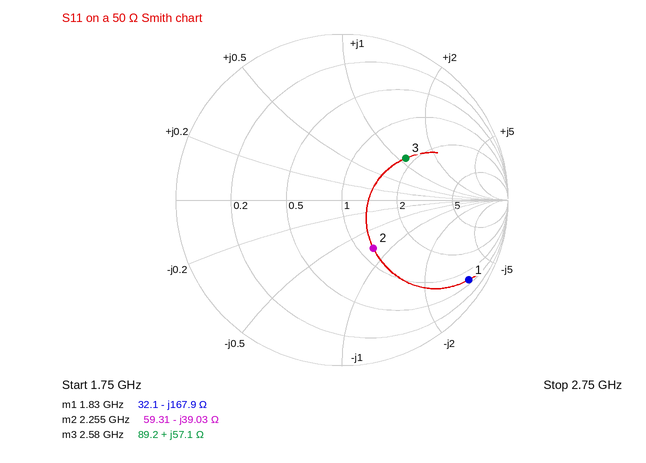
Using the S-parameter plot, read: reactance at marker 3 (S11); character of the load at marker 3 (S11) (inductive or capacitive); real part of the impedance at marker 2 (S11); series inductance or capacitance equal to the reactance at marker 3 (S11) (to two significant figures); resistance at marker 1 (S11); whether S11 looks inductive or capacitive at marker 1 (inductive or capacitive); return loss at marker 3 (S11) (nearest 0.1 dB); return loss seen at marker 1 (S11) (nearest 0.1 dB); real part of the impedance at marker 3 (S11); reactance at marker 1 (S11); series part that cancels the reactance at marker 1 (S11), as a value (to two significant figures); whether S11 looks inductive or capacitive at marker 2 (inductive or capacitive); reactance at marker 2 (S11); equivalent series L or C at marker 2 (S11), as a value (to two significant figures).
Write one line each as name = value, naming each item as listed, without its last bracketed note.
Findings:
reactance at marker 3 = +57.1 Ω
character of the load at marker 3 (S11) = inductive
real part of the impedance at marker 2 = 59.31 Ω
series inductance or capacitance equal to the reactance at marker 3 (S11) = 3.5 nH
resistance at marker 1 = 32.1 Ω
whether S11 looks inductive or capacitive at marker 1 = capacitive
return loss at marker 3 (S11) = 6.7 dB
return loss seen at marker 1 (S11) = 0.9 dB
real part of the impedance at marker 3 = 89.2 Ω
reactance at marker 1 = -167.9 Ω
series part that cancels the reactance at marker 1 (S11), as a value = 15 nH
whether S11 looks inductive or capacitive at marker 2 = capacitive
reactance at marker 2 = -39.03 Ω
equivalent series L or C at marker 2 (S11), as a value = 1.8 pF
